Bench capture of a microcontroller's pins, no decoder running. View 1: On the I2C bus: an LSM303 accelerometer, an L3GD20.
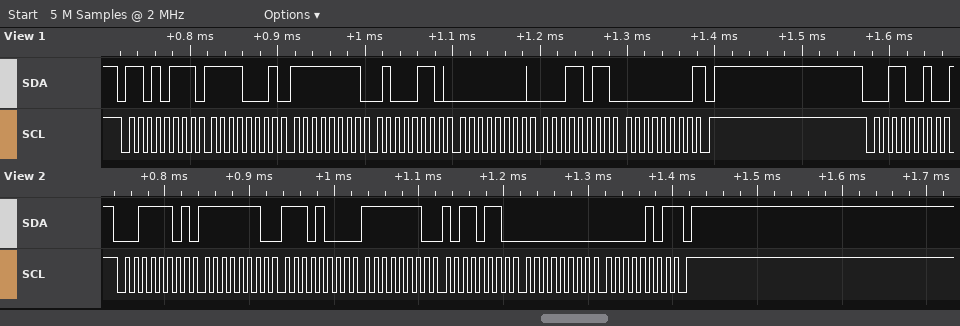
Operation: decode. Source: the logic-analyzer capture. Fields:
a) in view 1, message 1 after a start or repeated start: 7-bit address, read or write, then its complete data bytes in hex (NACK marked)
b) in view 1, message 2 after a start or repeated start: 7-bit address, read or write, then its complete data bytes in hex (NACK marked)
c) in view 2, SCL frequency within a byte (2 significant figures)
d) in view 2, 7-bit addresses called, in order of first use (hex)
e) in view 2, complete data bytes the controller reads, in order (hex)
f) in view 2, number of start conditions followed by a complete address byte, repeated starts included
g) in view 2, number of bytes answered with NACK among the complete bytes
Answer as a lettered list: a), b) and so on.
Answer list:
a) 0x6B read: F1 FF 46 00 1B 00 NACK
b) 0x19 write
c) 100 kHz
d) 0x1E
e) FE E8 FE B6 00 05
f) 1
g) 1
